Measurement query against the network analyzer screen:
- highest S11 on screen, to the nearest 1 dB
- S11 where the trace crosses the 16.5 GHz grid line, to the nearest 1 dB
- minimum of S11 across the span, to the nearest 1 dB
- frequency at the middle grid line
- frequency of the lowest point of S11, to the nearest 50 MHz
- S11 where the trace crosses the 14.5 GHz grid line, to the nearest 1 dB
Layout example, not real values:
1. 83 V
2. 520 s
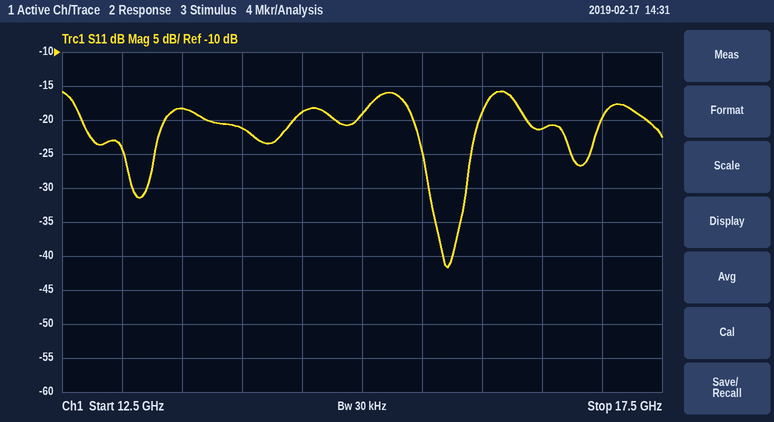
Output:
1. -16 dB
2. -21 dB
3. -42 dB
4. 15 GHz
5. 15.70 GHz
6. -19 dB
